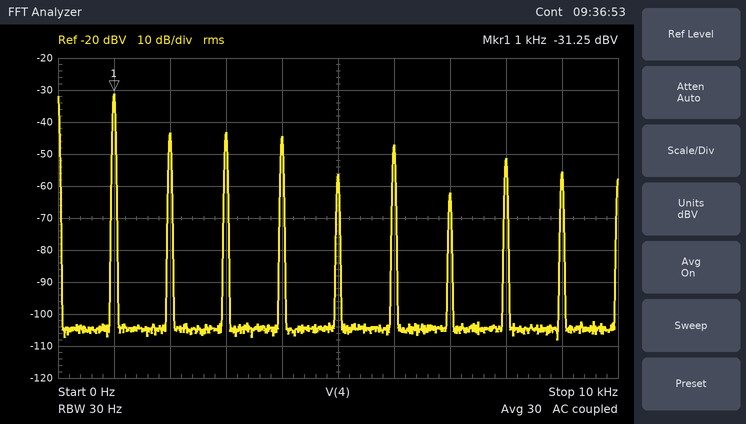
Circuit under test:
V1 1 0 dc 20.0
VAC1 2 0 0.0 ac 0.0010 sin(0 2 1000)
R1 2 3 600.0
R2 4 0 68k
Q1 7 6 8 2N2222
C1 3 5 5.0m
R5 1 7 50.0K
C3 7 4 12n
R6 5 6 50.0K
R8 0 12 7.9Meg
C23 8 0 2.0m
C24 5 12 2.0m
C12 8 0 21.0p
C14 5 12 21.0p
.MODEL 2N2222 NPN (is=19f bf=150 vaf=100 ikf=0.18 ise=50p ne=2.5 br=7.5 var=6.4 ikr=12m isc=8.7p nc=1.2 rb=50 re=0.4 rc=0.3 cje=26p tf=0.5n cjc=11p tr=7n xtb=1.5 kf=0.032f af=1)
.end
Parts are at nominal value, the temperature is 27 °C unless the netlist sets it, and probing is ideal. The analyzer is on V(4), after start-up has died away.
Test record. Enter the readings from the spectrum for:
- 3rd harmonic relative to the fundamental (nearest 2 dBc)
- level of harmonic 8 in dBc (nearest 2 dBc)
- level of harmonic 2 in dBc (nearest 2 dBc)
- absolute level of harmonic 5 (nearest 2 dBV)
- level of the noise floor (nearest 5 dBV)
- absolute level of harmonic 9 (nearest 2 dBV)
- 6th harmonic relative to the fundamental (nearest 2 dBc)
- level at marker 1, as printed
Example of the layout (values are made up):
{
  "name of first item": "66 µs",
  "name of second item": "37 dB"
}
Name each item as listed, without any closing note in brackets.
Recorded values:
{
  "3rd harmonic relative to the fundamental": "-12 dBc",
  "level of harmonic 8 in dBc": "-20 dBc",
  "level of harmonic 2 in dBc": "-12 dBc",
  "absolute level of harmonic 5": "-56 dBV",
  "level of the noise floor": "-105 dBV",
  "absolute level of harmonic 9": "-56 dBV",
  "6th harmonic relative to the fundamental": "-16 dBc",
  "level at marker 1, as printed": "-31.25 dBV"
}
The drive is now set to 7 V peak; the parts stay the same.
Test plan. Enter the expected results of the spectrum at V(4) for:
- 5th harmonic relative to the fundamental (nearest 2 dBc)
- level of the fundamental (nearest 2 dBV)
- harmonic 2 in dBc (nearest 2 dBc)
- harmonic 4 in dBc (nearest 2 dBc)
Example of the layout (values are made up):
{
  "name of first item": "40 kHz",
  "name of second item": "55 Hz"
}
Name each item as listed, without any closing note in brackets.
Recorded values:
{
  "5th harmonic relative to the fundamental": "-14 dBc",
  "level of the fundamental": "-32 dBV",
  "harmonic 2 in dBc": "-24 dBc",
  "harmonic 4 in dBc": "-22 dBc"
}
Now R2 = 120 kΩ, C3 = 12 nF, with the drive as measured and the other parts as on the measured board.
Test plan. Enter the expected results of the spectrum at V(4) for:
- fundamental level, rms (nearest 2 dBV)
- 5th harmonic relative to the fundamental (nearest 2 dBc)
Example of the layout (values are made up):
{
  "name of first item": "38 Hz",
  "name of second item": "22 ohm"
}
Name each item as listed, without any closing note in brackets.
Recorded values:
{
  "fundamental level, rms": "-30 dBV",
  "5th harmonic relative to the fundamental": "-24 dBc"
}
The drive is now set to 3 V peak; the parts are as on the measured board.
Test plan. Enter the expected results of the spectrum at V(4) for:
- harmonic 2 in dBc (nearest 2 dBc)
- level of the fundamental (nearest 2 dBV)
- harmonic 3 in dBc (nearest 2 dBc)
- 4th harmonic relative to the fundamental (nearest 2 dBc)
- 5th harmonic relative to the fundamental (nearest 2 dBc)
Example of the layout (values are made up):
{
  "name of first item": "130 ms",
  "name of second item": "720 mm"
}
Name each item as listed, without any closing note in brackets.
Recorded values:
{
  "harmonic 2 in dBc": "-16 dBc",
  "level of the fundamental": "-32 dBV",
  "harmonic 3 in dBc": "-10 dBc",
  "4th harmonic relative to the fundamental": "-16 dBc",
  "5th harmonic relative to the fundamental": "-18 dBc"
}
